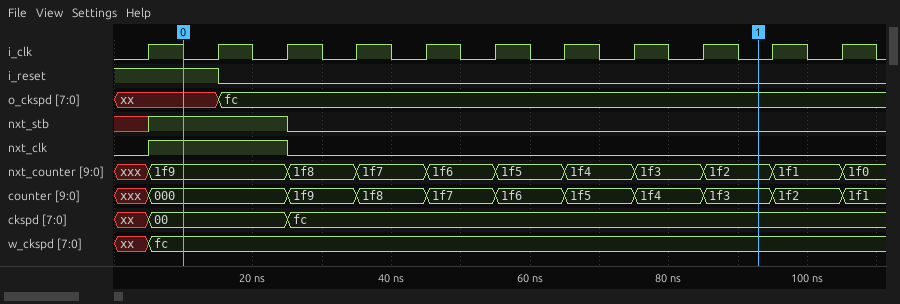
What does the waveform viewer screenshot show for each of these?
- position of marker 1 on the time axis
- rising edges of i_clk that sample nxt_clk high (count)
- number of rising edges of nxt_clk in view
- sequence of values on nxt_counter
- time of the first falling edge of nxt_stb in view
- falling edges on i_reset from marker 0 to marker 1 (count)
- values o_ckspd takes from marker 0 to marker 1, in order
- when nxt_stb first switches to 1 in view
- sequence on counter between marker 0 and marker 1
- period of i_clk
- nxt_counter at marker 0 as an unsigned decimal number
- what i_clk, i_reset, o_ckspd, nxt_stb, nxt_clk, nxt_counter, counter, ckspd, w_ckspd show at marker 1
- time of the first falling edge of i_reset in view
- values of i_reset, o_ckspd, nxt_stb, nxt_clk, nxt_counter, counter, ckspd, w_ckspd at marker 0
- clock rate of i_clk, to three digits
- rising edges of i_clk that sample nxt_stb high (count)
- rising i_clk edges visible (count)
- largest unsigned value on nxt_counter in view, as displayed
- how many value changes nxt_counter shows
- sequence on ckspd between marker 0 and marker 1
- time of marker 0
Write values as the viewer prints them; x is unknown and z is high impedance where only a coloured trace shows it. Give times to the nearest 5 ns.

95 ns
2
1
xxx, 1f9, 1f8, 1f7, 1f6, 1f5, 1f4, 1f3, 1f2, 1f1, 1f0
25 ns
1
xx, fc
5 ns
000, 1f9, 1f8, 1f7, 1f6, 1f5, 1f4, 1f3
10 ns
505
i_clk=0, i_reset=0, o_ckspd=fc, nxt_stb=0, nxt_clk=0, nxt_counter=1f2, counter=1f3, ckspd=fc, w_ckspd=fc
15 ns
i_reset=1, o_ckspd=xx, nxt_stb=1, nxt_clk=1, nxt_counter=1f9, counter=000, ckspd=00, w_ckspd=fc
100 MHz
2
11
1f9
10
00, fc
10 ns
